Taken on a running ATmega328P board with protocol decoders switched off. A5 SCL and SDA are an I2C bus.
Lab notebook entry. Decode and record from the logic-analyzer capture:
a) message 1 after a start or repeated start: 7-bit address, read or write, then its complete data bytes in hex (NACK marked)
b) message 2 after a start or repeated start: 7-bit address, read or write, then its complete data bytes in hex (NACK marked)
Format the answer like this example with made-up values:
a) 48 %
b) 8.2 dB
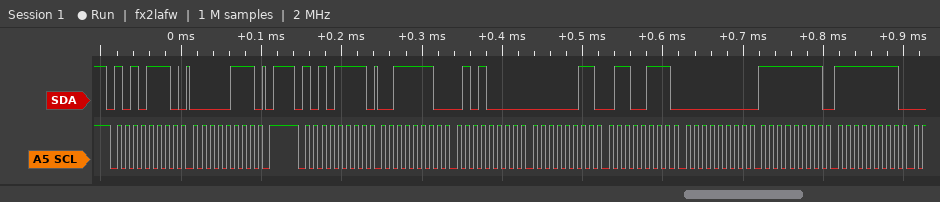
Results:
a) 0x57 write: 07
b) 0x57 read: 3E 50 03 67 00 FF FF
